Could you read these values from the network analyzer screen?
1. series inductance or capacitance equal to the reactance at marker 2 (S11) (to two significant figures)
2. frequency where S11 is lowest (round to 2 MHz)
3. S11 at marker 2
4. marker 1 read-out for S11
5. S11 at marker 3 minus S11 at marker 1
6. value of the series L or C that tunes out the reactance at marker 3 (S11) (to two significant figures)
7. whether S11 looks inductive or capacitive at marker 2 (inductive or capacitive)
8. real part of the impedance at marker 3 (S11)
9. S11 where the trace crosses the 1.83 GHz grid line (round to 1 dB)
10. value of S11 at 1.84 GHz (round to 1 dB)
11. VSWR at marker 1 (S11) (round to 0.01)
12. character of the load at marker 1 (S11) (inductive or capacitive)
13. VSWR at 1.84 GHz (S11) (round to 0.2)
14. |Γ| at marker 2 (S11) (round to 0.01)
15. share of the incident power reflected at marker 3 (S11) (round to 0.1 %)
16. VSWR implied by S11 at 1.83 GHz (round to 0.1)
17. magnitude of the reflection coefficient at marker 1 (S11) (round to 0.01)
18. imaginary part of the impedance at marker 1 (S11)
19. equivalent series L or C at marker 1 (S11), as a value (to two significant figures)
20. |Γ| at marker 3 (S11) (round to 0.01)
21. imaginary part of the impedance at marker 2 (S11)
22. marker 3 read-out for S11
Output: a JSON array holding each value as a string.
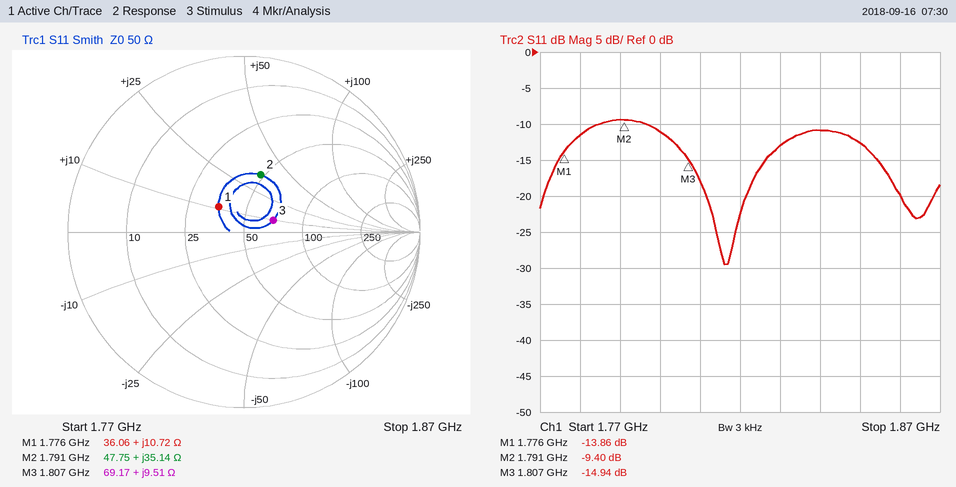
["3.1 nH", "1.816 GHz", "-9.40 dB", "-13.86 dB", "-1.08 dB", "9.3 pF", "inductive", "69.17 Ω", "-13 dB", "-11 dB", "1.51", "inductive", "1.8", "0.34", "3.2 %", "1.6", "0.20", "+10.72 Ω", "960 pH", "0.18", "+35.14 Ω", "-14.94 dB"]
